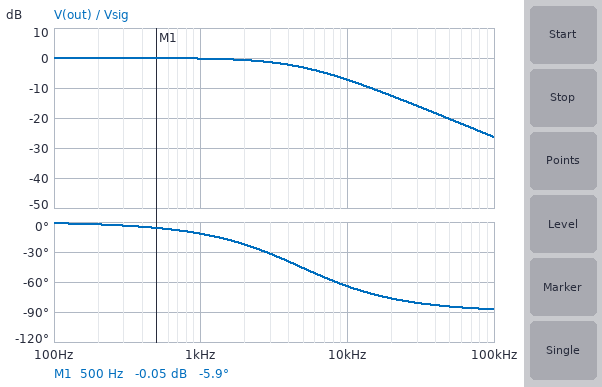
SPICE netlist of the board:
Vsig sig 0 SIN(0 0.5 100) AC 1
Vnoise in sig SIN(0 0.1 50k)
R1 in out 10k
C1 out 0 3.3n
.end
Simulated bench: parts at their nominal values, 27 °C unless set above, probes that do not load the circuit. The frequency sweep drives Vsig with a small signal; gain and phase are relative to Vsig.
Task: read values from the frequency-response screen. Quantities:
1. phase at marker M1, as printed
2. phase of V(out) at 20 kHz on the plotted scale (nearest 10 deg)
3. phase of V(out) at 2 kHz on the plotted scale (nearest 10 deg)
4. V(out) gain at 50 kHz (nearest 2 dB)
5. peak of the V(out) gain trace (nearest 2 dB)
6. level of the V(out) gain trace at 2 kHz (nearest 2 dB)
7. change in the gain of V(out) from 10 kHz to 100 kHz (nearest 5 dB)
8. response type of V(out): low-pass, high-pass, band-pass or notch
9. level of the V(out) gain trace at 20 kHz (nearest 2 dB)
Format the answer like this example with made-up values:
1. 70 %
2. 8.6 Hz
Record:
1. -5.9 deg
2. -80 deg
3. -20 deg
4. -20 dB
5. 0 dB
6. 0 dB
7. -20 dB
8. low-pass
9. -12 dB
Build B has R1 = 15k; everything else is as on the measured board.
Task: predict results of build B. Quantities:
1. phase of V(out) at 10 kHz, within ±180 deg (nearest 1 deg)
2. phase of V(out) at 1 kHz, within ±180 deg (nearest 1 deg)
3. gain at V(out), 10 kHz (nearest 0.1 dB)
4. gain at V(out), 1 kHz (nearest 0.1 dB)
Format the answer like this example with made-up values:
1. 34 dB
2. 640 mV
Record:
1. -72 deg
2. -17 deg
3. -10.3 dB
4. -0.4 dB
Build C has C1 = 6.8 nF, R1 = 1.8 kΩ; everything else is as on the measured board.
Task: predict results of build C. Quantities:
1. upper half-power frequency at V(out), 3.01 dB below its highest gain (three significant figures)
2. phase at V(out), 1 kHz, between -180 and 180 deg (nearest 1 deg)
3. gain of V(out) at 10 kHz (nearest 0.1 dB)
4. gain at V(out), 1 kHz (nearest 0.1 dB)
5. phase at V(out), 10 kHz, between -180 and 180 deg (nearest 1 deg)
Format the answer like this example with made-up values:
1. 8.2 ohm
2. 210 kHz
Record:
1. 13.0 kHz
2. -4 deg
3. -2.0 dB
4. 0 dB
5. -38 deg
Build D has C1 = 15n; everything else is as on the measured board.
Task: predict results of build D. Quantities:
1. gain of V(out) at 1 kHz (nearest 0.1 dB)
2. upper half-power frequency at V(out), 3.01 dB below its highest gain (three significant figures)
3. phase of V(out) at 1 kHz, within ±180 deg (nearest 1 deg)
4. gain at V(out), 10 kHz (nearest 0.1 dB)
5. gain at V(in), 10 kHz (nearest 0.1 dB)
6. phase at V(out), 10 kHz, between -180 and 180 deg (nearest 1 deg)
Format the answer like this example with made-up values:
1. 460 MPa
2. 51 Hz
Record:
1. -2.8 dB
2. 1.06 kHz
3. -43 deg
4. -19.5 dB
5. 0 dB
6. -84 deg
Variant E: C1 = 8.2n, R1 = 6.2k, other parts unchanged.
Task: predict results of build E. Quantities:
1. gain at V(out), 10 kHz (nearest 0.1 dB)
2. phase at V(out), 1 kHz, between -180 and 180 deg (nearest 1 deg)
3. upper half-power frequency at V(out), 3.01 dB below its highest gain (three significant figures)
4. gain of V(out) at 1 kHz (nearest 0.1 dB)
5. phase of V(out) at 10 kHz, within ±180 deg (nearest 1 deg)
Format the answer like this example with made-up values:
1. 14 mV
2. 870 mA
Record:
1. -10.5 dB
2. -18 deg
3. 3.13 kHz
4. -0.4 dB
5. -73 deg
